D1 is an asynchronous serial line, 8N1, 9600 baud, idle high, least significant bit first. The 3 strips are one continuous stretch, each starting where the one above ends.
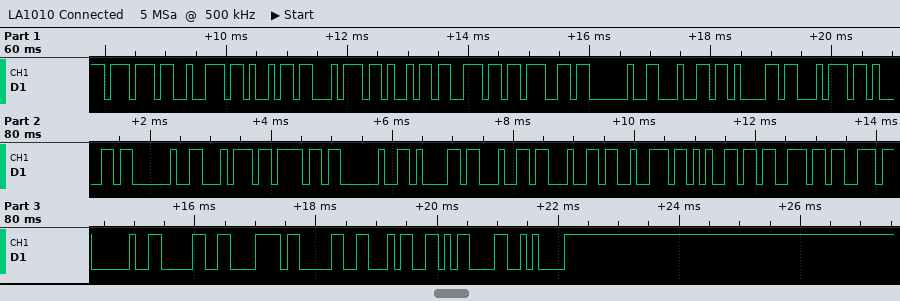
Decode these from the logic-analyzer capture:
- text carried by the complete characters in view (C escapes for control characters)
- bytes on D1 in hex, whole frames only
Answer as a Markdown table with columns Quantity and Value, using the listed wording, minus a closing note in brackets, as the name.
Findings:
| Quantity | Value |
|---|---|
| text carried by the complete characters in view | "writing data to address 0x04\r\n" |
| bytes on D1 in hex, whole frames only | 77 72 69 74 69 6E 67 20 64 61 74 61 20 74 6F 20 61 64 64 72 65 73 73 20 30 78 30 34 0D 0A |
